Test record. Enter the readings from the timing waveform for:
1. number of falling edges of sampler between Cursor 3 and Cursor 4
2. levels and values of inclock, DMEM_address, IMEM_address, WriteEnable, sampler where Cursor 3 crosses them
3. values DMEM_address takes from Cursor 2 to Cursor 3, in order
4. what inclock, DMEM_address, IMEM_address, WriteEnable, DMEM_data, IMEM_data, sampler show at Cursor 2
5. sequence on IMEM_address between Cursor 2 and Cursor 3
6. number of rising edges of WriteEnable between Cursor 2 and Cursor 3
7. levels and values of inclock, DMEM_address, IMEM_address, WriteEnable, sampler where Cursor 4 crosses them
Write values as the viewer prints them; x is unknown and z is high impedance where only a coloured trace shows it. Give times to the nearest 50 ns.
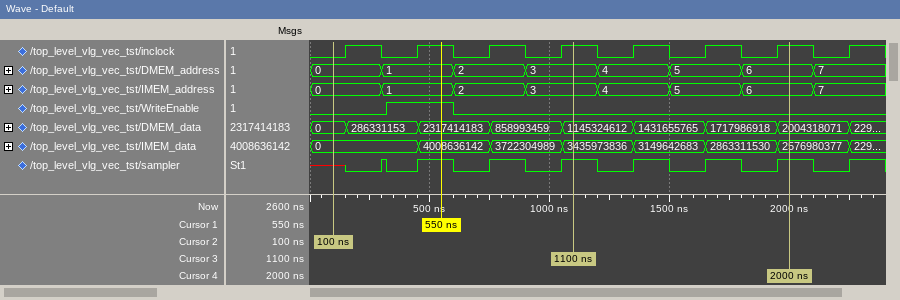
3
inclock=1, DMEM_address=3, IMEM_address=3, WriteEnable=0, sampler=1
0, 1, 2, 3
inclock=0, DMEM_address=0, IMEM_address=0, WriteEnable=0, DMEM_data=0, IMEM_data=0, sampler=x
0, 1, 2, 3
1
inclock=1, DMEM_address=6, IMEM_address=6, WriteEnable=0, sampler=1
